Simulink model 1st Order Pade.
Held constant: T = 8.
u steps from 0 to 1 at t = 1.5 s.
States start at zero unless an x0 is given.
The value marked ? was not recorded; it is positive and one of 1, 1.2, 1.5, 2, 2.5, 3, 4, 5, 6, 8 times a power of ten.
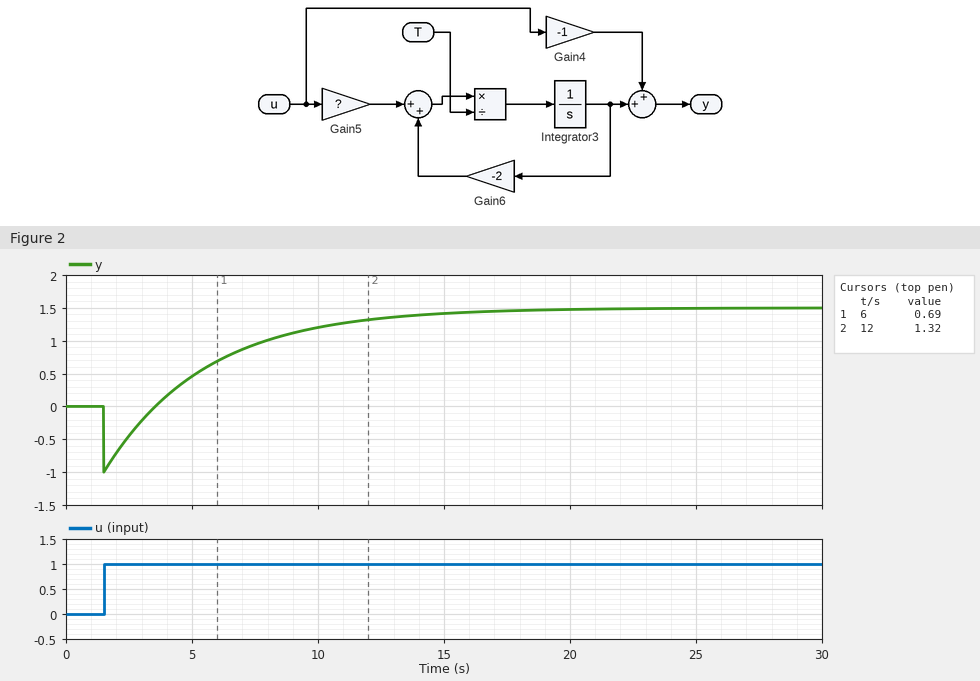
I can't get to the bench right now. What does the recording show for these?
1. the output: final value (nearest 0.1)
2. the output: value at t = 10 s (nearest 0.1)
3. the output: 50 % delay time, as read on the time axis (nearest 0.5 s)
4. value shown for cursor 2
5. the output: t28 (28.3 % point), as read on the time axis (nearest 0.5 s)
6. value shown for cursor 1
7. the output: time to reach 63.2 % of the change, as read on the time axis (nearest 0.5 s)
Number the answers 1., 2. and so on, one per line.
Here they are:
1. 1.5
2. 1.2
3. 6.5 s
4. 1.32
5. 5.0 s
6. 0.69
7. 7.5 s
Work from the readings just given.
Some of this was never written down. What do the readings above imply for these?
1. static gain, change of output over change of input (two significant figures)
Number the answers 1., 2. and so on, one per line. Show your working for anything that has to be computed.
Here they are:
1. (1.5 - 0) / (1 - 0) = 1.5
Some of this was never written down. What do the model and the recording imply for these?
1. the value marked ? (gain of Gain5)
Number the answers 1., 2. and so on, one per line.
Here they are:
1. 5
